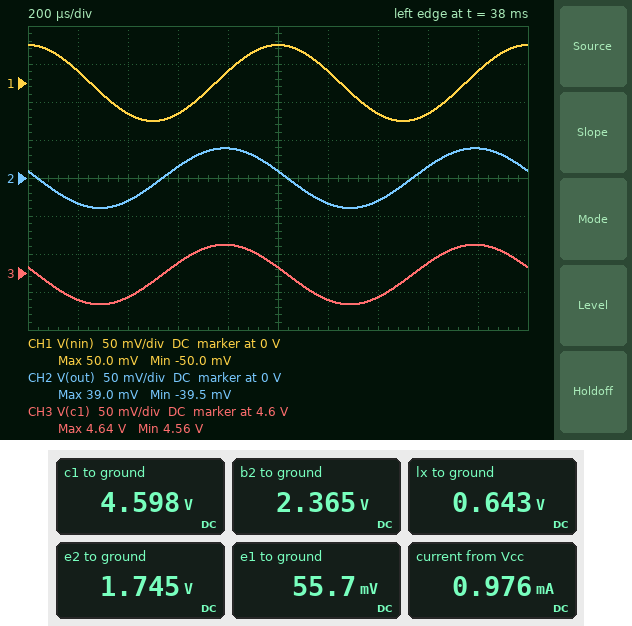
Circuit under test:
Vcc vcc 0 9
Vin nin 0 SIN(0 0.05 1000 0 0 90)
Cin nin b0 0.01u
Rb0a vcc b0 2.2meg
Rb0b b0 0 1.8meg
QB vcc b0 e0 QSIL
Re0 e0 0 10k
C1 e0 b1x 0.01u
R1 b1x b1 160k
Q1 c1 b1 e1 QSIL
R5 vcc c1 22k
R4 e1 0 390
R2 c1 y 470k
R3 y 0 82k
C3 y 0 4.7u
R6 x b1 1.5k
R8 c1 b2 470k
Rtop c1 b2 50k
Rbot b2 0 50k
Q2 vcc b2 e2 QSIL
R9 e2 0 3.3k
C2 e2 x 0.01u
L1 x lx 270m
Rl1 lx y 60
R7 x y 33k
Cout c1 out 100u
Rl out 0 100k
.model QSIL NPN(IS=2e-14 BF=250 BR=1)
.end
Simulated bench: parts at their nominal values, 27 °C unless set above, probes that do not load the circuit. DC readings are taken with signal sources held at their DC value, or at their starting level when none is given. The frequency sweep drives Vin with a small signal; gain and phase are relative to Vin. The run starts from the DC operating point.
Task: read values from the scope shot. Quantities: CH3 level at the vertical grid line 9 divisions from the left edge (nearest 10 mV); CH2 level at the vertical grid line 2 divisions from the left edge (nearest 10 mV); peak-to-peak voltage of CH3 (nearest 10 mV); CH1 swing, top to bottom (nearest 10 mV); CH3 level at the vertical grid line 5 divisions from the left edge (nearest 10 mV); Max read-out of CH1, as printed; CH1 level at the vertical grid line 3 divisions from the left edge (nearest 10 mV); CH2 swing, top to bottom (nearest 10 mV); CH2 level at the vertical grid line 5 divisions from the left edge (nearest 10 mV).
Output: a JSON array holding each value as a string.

["4.64 V", "-30 mV", "80 mV", "100 mV", "4.61 V", "50.0 mV", "-40 mV", "80 mV", "10 mV"]
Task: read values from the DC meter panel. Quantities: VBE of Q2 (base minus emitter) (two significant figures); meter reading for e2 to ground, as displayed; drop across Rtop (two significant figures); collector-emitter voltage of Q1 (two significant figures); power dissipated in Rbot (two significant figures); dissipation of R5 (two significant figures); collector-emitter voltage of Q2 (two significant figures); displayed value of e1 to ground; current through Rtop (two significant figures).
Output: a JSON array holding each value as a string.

["620 mV", "1.745 V", "2.2 V", "4.5 V", "110 µW", "880 µW", "7.3 V", "55.7 mV", "45 µA"]
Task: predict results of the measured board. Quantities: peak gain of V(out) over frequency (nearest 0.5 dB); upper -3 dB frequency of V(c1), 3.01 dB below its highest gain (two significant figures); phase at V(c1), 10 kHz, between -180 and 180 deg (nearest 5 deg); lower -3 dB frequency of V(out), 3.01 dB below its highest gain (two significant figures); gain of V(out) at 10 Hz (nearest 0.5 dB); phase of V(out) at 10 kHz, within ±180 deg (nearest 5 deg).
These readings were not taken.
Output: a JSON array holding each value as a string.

["9.0 dB", "890 Hz", "135 deg", "800 Hz", "-33.0 dB", "135 deg"]
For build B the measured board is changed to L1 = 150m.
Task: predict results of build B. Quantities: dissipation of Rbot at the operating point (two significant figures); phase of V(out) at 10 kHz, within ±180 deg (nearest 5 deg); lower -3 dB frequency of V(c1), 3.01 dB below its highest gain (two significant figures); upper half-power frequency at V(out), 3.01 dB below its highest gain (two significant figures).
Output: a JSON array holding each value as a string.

["110 µW", "130 deg", "1.1 kHz", "1.2 kHz"]
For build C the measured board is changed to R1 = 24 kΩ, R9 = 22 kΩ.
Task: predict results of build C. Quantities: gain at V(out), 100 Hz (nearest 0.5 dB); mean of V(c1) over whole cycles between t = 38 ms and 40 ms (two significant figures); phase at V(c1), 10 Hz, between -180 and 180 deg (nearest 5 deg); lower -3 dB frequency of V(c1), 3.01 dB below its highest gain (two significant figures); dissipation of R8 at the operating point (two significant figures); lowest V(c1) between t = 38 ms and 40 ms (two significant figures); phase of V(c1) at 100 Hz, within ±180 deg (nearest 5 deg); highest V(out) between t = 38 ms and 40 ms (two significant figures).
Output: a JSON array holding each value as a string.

["-12.5 dB", "4.6 V", "-75 deg", "760 Hz", "10 µW", "4.4 V", "-90 deg", "190 mV"]
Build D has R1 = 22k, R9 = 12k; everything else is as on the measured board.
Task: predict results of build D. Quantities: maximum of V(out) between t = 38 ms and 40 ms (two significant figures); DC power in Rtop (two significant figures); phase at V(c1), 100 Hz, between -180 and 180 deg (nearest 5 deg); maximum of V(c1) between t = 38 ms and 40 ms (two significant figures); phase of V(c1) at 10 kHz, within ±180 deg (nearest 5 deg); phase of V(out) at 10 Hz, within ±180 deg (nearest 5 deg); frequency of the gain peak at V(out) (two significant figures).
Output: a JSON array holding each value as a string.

["200 mV", "97 µW", "-90 deg", "4.8 V", "140 deg", "-75 deg", "830 Hz"]
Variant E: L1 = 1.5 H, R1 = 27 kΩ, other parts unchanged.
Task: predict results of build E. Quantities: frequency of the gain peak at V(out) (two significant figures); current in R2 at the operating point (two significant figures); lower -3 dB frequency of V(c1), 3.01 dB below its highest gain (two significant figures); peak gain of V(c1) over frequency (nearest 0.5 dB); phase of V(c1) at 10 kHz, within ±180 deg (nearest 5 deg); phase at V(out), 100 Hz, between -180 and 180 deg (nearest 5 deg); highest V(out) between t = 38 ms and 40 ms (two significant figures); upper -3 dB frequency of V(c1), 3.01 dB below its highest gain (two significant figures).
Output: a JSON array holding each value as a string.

["350 Hz", "8.4 µA", "320 Hz", "19.0 dB", "140 deg", "-65 deg", "54 mV", "390 Hz"]
